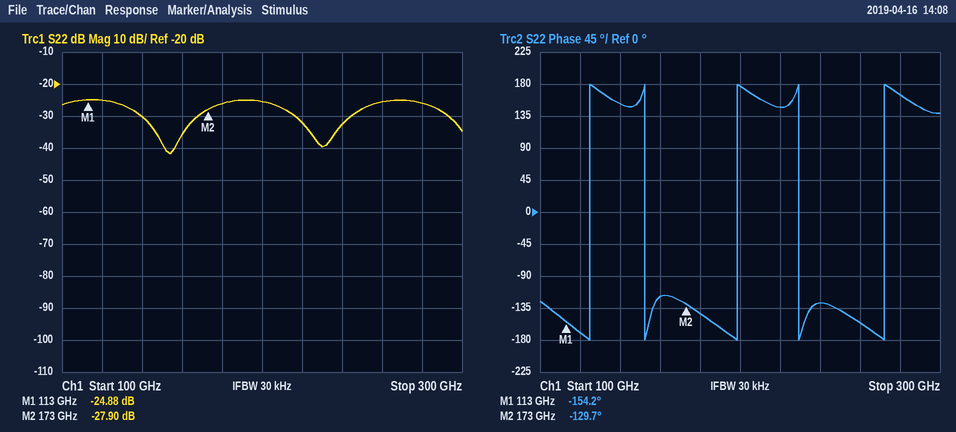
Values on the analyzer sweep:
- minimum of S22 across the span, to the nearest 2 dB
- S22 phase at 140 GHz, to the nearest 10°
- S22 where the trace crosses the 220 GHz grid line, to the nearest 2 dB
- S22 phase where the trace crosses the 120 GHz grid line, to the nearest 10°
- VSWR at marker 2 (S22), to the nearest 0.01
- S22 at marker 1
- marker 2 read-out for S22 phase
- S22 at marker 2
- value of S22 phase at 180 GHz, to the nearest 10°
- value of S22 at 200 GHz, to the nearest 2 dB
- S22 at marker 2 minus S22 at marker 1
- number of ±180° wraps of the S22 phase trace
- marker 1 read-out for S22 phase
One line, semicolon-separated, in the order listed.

-42 dB; 150°; -32 dB; -170°; 1.08; -24.88 dB; -129.7°; -27.90 dB; -140°; -26 dB; -3.02 dB; 5; -154.2°
